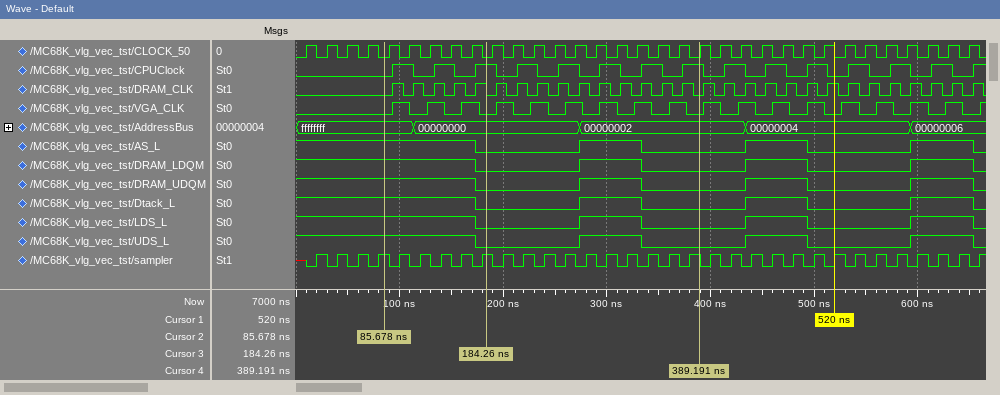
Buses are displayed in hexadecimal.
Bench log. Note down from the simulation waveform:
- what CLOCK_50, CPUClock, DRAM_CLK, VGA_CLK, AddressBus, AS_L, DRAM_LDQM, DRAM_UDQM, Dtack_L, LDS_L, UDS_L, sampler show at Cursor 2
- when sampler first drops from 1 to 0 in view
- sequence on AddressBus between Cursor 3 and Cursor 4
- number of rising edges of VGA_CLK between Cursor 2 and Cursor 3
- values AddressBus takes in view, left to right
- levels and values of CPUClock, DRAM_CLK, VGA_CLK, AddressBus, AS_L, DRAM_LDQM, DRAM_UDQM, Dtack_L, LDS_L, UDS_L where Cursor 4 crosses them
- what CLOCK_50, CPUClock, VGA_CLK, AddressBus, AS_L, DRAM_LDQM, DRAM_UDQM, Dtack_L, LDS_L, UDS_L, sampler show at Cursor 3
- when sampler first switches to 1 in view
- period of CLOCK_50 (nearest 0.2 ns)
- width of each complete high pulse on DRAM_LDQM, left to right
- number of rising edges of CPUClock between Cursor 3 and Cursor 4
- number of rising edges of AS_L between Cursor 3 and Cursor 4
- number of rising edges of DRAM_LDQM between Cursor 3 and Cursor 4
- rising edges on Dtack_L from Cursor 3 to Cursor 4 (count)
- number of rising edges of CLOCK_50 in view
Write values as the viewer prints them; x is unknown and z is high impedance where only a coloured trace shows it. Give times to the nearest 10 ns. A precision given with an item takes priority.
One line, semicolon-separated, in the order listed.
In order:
CLOCK_50=0, CPUClock=0, DRAM_CLK=0, VGA_CLK=0, AddressBus=ffffffff, AS_L=1, DRAM_LDQM=1, DRAM_UDQM=1, Dtack_L=1, LDS_L=1, UDS_L=1, sampler=1; 30 ns; 00000000, 00000002; 3; ffffffff, 00000000, 00000002, 00000004, 00000006; CPUClock=1, DRAM_CLK=0, VGA_CLK=0, AddressBus=00000002, AS_L=0, DRAM_LDQM=0, DRAM_UDQM=0, Dtack_L=0, LDS_L=0, UDS_L=0; CLOCK_50=0, CPUClock=1, VGA_CLK=0, AddressBus=00000000, AS_L=0, DRAM_LDQM=0, DRAM_UDQM=0, Dtack_L=0, LDS_L=0, UDS_L=0, sampler=1; 20 ns; 20 ns; 60 ns, 60 ns, 60 ns; 5; 1; 1; 1; 33
